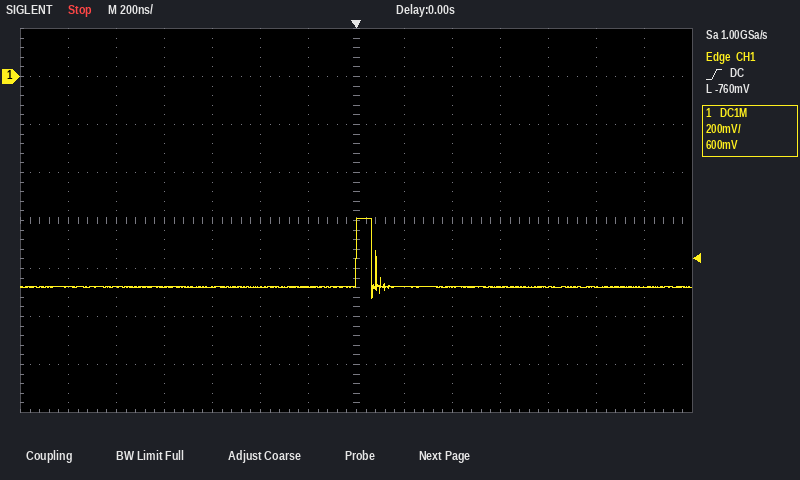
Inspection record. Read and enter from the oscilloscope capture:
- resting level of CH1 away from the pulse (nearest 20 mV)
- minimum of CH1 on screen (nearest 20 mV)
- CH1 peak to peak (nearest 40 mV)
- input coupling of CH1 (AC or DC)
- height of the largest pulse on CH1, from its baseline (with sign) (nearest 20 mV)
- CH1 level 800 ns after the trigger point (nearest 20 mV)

-880 mV
-920 mV
320 mV
DC
+280 mV
-880 mV
